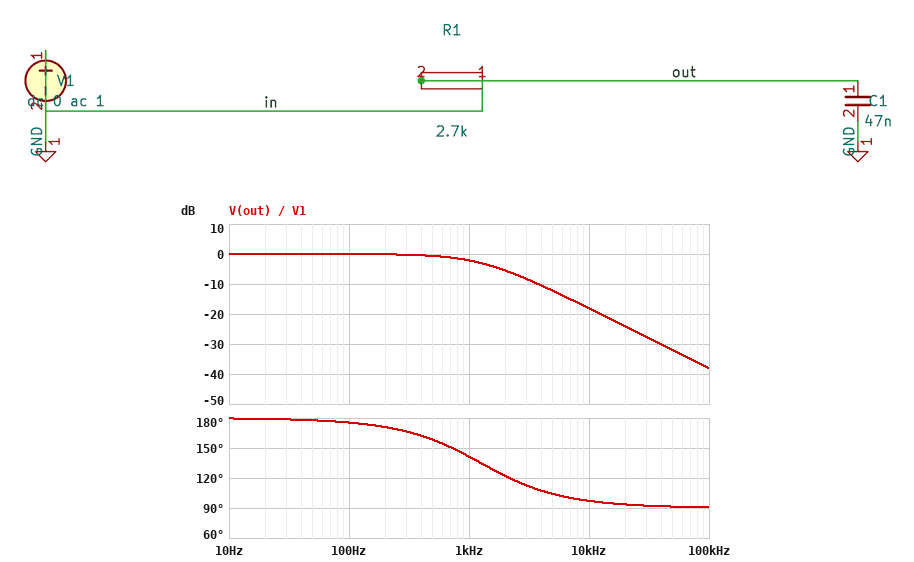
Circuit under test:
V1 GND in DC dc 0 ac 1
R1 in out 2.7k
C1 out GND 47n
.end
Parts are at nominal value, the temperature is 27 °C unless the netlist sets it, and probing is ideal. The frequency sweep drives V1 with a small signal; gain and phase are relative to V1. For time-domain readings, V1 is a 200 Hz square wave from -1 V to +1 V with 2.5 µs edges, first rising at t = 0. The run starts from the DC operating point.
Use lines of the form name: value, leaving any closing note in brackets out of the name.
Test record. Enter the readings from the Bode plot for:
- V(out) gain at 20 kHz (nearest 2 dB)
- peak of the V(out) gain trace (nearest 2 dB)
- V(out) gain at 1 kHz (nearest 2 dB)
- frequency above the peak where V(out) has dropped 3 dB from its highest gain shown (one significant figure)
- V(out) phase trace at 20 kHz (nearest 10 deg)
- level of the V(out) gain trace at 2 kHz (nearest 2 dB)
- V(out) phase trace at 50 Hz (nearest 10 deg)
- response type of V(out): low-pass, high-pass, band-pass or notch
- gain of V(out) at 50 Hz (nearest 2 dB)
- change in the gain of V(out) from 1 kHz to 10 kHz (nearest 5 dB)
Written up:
V(out) gain at 20 kHz: -24 dB
peak of the V(out) gain trace: 0 dB
V(out) gain at 1 kHz: -2 dB
frequency above the peak where V(out) has dropped 3 dB from its highest gain shown: 1 kHz
V(out) phase trace at 20 kHz: 90 deg
level of the V(out) gain trace at 2 kHz: -6 dB
V(out) phase trace at 50 Hz: 180 deg
response type of V(out): low-pass, high-pass, band-pass or notch: low-pass
gain of V(out) at 50 Hz: 0 dB
change in the gain of V(out) from 1 kHz to 10 kHz: -15 dB
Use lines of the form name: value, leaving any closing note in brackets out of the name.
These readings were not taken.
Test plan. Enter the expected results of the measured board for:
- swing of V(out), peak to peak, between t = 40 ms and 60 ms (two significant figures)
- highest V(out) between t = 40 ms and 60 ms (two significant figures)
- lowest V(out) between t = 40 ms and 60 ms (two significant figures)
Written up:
swing of V(out), peak to peak, between t = 40 ms and 60 ms: 2.0 V
highest V(out) between t = 40 ms and 60 ms: 1.0 V
lowest V(out) between t = 40 ms and 60 ms: -1.0 V
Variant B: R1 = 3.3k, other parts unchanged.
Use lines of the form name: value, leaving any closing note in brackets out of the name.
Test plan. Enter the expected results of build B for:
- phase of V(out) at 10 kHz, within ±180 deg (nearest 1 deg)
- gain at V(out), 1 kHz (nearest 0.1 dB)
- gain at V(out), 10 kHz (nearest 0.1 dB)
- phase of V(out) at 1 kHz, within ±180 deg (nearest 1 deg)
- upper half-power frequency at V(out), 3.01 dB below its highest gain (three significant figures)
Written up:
phase of V(out) at 10 kHz, within ±180 deg: 96 deg
gain at V(out), 1 kHz: -2.9 dB
gain at V(out), 10 kHz: -19.8 dB
phase of V(out) at 1 kHz, within ±180 deg: 136 deg
upper half-power frequency at V(out), 3.01 dB below its highest gain: 1.03 kHz
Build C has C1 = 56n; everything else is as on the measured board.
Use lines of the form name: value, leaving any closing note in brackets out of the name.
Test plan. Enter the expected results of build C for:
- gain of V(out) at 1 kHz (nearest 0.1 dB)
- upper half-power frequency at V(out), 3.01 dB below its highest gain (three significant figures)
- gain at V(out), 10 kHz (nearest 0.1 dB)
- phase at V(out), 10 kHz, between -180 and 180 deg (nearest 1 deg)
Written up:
gain of V(out) at 1 kHz: -2.8 dB
upper half-power frequency at V(out), 3.01 dB below its highest gain: 1.05 kHz
gain at V(out), 10 kHz: -19.6 dB
phase at V(out), 10 kHz, between -180 and 180 deg: 96 deg
